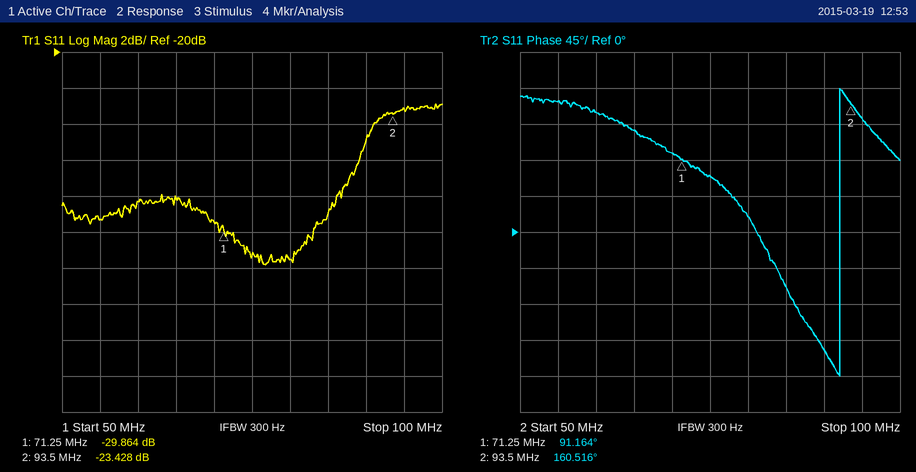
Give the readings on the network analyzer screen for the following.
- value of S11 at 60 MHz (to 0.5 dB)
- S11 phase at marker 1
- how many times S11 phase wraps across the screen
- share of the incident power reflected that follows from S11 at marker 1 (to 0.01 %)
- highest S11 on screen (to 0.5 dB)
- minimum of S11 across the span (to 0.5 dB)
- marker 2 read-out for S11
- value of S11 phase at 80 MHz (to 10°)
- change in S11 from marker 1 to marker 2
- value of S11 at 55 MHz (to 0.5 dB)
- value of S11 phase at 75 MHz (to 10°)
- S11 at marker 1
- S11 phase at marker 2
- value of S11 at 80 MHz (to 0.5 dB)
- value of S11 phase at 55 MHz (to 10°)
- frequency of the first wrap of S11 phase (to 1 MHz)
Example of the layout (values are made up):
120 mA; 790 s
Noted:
-28.5 dB; 91.164°; 1; 0.10 %; -23.0 dB; -32.0 dB; -23.428 dB; 20°; 6.436 dB; -29.5 dB; 70°; -29.864 dB; 160.516°; -31.5 dB; 160°; 92 MHz
